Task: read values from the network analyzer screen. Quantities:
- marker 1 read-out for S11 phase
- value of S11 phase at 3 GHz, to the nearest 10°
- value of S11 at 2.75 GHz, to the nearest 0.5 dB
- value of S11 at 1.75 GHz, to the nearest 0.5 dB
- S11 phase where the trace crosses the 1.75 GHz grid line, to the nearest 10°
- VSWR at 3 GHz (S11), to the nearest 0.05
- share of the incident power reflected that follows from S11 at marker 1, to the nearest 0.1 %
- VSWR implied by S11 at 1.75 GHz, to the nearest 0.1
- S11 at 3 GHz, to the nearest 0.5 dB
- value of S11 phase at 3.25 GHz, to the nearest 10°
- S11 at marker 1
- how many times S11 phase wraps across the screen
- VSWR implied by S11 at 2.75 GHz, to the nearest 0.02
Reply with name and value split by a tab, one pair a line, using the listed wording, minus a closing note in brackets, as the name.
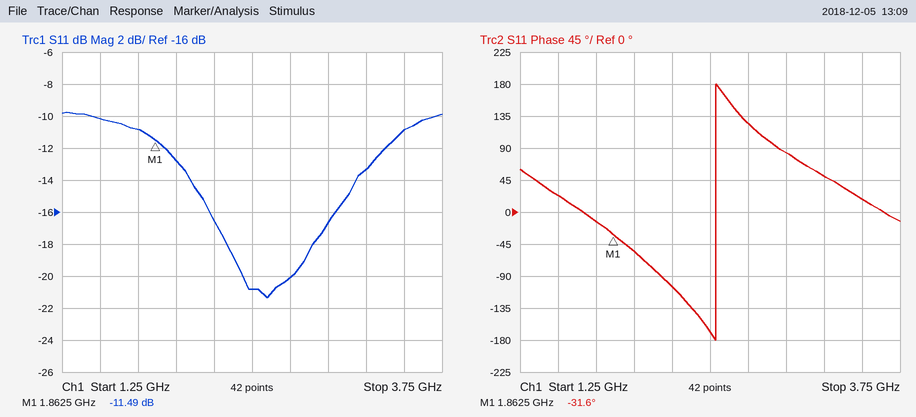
marker 1 read-out for S11 phase	-31.6°
value of S11 phase at 3 GHz, to the nearest 10°	80°
value of S11 at 2.75 GHz, to the nearest 0.5 dB	-20.0 dB
value of S11 at 1.75 GHz, to the nearest 0.5 dB	-11.0 dB
S11 phase where the trace crosses the 1.75 GHz grid line, to the nearest 10°	-10°
VSWR at 3 GHz (S11), to the nearest 0.05	1.35
share of the incident power reflected that follows from S11 at marker 1, to the nearest 0.1 %	7.1 %
VSWR implied by S11 at 1.75 GHz, to the nearest 0.1	1.8
S11 at 3 GHz, to the nearest 0.5 dB	-16.5 dB
value of S11 phase at 3.25 GHz, to the nearest 10°	50°
S11 at marker 1	-11.49 dB
how many times S11 phase wraps across the screen	1
VSWR implied by S11 at 2.75 GHz, to the nearest 0.02	1.22
